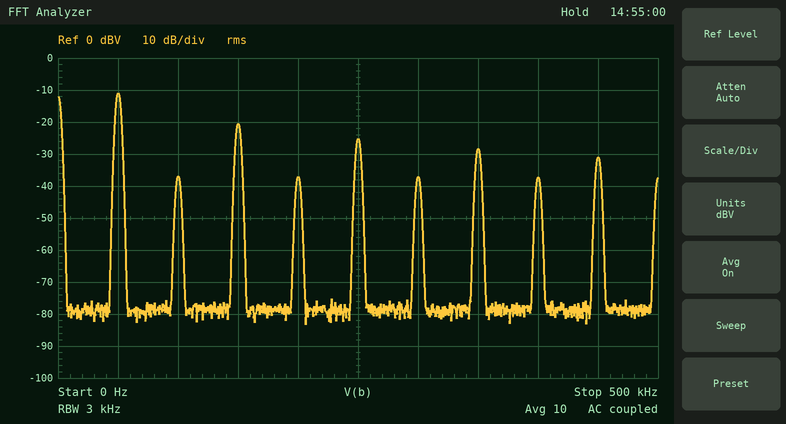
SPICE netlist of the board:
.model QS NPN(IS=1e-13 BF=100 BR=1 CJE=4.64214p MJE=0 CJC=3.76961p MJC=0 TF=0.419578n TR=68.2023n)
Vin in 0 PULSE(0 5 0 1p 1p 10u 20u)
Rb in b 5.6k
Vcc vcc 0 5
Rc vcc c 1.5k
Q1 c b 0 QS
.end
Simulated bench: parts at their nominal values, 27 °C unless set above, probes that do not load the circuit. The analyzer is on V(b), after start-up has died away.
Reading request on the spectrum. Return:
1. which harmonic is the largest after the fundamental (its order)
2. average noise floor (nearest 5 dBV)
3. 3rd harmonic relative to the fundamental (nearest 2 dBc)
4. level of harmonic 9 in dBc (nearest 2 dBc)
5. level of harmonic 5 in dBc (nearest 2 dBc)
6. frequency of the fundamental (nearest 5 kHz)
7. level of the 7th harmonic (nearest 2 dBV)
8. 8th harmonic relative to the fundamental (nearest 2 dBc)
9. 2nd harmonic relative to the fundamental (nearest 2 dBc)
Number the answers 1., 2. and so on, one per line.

1. 3
2. -80 dBV
3. -10 dBc
4. -20 dBc
5. -14 dBc
6. 50 kHz
7. -28 dBV
8. -26 dBc
9. -26 dBc
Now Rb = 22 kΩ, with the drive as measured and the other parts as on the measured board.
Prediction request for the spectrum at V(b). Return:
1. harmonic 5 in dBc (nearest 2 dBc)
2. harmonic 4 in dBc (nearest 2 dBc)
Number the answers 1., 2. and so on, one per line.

1. -16 dBc
2. -20 dBc
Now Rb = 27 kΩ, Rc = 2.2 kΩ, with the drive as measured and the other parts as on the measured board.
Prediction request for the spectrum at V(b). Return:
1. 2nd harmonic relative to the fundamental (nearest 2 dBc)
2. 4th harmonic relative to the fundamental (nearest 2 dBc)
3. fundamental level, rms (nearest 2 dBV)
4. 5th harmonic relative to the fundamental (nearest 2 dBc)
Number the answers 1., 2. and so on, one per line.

1. -18 dBc
2. -18 dBc
3. -12 dBV
4. -16 dBc
